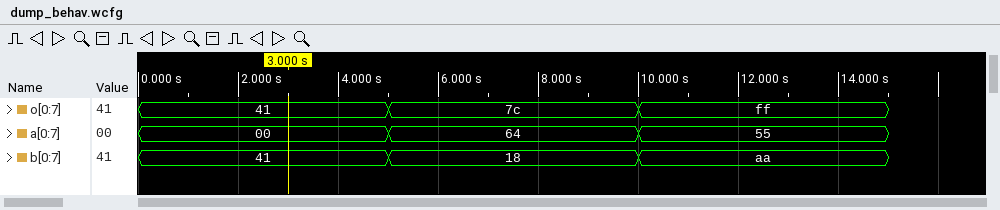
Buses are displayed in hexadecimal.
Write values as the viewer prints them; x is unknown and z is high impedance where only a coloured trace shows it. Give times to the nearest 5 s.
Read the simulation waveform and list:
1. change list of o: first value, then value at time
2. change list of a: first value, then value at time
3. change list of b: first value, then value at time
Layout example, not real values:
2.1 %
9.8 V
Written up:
41, 7c at 5 s, ff at 10 s
00, 64 at 5 s, 55 at 10 s
41, 18 at 5 s, aa at 10 s
